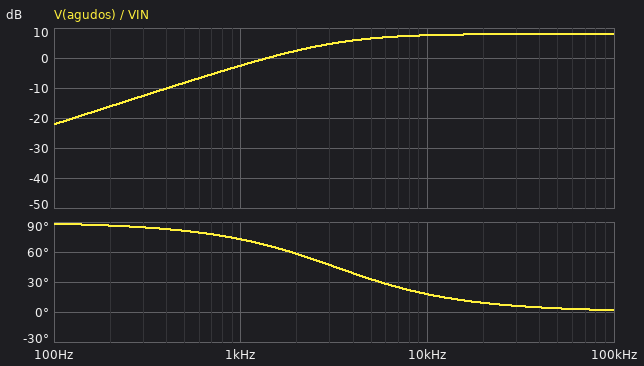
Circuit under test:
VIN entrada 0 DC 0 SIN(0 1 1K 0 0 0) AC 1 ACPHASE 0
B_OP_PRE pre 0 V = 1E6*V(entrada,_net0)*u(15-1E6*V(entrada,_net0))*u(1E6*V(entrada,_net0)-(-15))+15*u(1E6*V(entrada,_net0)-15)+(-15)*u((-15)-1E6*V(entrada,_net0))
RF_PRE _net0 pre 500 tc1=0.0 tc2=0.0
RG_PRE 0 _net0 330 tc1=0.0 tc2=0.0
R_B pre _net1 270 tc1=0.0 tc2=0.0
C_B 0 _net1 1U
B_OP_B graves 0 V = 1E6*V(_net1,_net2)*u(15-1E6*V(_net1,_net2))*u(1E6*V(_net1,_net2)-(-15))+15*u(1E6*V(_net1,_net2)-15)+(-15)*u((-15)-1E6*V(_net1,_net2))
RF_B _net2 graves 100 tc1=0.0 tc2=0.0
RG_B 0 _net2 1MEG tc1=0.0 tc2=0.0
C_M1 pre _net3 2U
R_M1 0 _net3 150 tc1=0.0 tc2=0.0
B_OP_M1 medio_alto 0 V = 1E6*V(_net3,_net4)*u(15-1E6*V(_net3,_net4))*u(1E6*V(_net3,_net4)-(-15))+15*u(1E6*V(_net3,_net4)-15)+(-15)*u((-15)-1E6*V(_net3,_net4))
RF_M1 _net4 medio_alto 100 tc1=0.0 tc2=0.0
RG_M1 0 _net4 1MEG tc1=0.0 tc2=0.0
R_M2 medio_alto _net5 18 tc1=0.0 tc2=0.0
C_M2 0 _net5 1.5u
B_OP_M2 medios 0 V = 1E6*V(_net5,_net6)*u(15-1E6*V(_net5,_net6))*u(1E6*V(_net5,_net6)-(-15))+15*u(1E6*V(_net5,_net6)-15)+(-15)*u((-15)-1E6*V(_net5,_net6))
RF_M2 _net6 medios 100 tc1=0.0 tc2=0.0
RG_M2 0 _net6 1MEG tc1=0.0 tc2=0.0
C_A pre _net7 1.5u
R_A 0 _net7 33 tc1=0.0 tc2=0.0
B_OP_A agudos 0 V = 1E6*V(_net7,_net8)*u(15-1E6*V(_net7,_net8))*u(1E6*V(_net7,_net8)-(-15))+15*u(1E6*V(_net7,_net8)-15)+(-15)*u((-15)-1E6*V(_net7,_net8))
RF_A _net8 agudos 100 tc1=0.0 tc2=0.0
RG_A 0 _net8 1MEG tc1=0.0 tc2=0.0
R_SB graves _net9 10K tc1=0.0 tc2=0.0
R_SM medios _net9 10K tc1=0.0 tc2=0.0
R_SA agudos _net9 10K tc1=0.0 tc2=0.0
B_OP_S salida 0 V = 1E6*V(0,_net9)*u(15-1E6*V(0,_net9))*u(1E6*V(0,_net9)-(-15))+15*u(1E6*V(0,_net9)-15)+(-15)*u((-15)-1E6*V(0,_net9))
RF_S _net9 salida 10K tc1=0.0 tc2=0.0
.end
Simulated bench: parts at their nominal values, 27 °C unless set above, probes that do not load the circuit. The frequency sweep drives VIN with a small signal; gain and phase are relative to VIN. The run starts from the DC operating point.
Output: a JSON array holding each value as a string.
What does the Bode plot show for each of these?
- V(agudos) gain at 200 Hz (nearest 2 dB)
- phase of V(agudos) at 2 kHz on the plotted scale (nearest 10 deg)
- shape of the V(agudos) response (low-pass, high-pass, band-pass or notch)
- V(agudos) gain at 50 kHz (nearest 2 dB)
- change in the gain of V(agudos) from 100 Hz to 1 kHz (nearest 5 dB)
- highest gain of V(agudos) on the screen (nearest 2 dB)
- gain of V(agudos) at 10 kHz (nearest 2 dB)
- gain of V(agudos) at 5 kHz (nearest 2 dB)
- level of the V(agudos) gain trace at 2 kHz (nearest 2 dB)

["-16 dB", "60 deg", "high-pass", "8 dB", "20 dB", "8 dB", "8 dB", "6 dB", "2 dB"]
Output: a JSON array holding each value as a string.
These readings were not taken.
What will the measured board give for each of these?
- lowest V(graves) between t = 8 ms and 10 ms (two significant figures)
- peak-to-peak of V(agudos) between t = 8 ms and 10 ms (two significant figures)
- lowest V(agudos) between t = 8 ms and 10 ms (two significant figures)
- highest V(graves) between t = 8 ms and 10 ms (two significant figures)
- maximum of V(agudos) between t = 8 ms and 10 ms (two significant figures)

["-1.3 V", "1.5 V", "-750 mV", "1.3 V", "750 mV"]
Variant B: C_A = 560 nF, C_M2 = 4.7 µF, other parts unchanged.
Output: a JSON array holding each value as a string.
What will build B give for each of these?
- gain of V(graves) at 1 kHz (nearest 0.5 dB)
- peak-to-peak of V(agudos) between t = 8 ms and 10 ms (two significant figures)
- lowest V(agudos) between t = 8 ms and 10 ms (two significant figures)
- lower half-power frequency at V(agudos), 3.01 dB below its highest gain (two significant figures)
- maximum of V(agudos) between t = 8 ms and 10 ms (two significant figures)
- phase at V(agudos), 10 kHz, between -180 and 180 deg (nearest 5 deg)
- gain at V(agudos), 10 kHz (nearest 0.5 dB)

["2.0 dB", "580 mV", "-290 mV", "8.6 kHz", "290 mV", "40 deg", "5.5 dB"]
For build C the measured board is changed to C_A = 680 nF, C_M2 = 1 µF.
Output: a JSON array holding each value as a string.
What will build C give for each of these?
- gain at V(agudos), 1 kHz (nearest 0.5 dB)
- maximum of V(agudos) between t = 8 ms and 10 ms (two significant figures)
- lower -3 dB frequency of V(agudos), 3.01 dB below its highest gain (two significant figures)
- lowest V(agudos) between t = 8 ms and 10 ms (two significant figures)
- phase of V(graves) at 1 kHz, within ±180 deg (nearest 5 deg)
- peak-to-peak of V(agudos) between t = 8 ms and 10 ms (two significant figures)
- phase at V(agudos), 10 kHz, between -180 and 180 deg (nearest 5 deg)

["-9.0 dB", "350 mV", "7.1 kHz", "-350 mV", "-60 deg", "700 mV", "35 deg"]
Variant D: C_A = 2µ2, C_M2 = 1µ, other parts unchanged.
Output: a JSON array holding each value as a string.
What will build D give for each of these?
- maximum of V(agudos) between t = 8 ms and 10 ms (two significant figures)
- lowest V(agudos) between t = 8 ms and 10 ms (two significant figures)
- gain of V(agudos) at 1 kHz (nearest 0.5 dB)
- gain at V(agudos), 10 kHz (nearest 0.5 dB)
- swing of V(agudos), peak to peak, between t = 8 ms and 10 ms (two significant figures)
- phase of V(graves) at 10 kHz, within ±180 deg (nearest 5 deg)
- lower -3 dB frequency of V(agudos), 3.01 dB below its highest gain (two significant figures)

["1.0 V", "-1.0 V", "0.5 dB", "8.0 dB", "2.1 V", "-85 deg", "2.2 kHz"]
